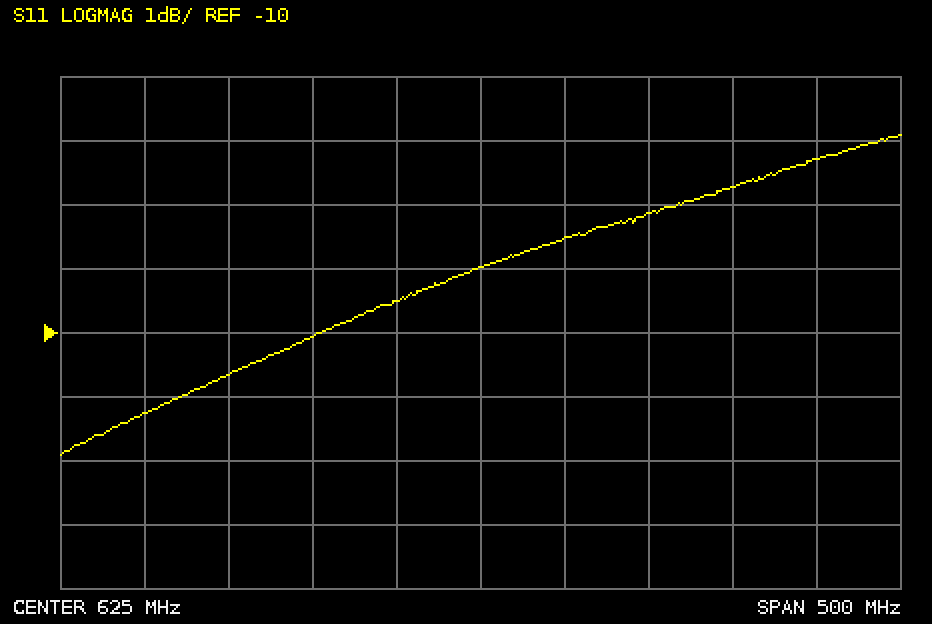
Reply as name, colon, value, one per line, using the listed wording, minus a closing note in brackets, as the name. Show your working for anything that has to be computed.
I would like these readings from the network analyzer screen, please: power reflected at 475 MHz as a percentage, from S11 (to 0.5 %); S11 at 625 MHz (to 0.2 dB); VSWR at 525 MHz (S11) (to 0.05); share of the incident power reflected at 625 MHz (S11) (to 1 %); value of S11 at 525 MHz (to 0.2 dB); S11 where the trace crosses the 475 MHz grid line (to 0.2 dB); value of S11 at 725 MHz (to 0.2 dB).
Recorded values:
power reflected at 475 MHz as a percentage, from S11: 10^(-10.6/10) ≈ 8.71 %, so 8.5 % to the nearest 0.5 %
S11 at 625 MHz: -9.0 dB
VSWR at 525 MHz (S11): |Γ| = 10^(-10/20) = 0.3162; VSWR = (1 + 0.3162)/(1 − 0.3162) ≈ 1.92, so 1.90 to the nearest 0.05
share of the incident power reflected at 625 MHz (S11): 10^(-9/10) ≈ 13 %
value of S11 at 525 MHz: -10.0 dB
S11 where the trace crosses the 475 MHz grid line: -10.6 dB
value of S11 at 725 MHz: -8.2 dB
